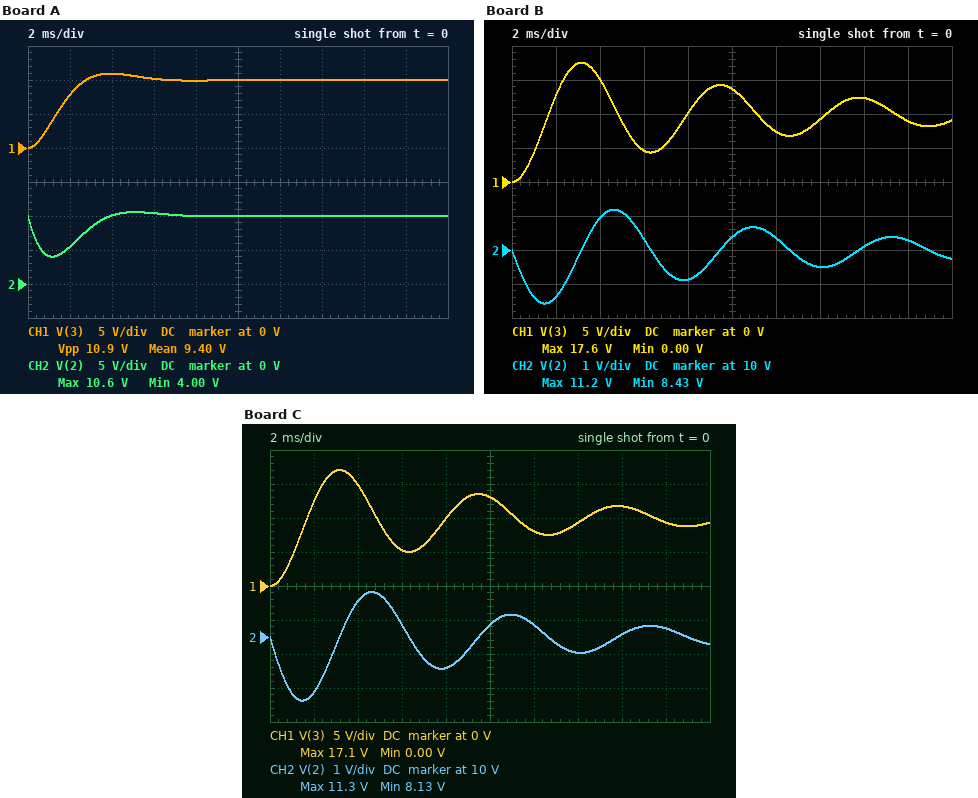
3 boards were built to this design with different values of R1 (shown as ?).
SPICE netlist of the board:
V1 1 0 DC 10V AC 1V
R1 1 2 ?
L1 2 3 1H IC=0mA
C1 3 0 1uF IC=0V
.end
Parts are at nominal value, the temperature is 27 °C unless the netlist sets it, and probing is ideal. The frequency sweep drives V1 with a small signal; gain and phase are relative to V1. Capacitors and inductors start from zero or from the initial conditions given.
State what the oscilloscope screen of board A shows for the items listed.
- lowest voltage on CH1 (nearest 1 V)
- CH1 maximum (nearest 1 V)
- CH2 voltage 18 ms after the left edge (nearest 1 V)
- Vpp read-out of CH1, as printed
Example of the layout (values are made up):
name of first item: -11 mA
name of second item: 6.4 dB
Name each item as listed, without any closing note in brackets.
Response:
lowest voltage on CH1: 0 V
CH1 maximum: 11 V
CH2 voltage 18 ms after the left edge: 10 V
Vpp read-out of CH1, as printed: 10.9 V
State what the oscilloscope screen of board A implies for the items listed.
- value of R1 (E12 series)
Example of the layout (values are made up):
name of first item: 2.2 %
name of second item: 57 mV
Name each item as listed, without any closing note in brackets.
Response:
value of R1: 1.2 kΩ
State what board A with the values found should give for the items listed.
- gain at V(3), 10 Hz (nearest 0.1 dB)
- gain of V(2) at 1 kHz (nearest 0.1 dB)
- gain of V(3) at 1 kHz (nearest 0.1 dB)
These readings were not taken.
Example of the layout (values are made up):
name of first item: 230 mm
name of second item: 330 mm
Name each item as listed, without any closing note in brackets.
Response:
gain at V(3), 10 Hz: 0 dB
gain of V(2) at 1 kHz: -0.2 dB
gain of V(3) at 1 kHz: -31.9 dB
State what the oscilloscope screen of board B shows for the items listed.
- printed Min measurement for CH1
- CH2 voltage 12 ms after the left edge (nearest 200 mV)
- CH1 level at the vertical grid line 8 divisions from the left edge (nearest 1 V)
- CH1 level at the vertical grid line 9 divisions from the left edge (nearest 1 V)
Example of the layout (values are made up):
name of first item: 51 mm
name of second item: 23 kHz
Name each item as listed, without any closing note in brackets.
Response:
printed Min measurement for CH1: 0.00 V
CH2 voltage 12 ms after the left edge: 10.4 V
CH1 level at the vertical grid line 8 divisions from the left edge: 12 V
CH1 level at the vertical grid line 9 divisions from the left edge: 9 V
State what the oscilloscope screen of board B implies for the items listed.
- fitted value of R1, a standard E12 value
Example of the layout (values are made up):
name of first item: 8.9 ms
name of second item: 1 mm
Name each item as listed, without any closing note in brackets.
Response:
fitted value of R1, a standard E12 value: 180 Ω
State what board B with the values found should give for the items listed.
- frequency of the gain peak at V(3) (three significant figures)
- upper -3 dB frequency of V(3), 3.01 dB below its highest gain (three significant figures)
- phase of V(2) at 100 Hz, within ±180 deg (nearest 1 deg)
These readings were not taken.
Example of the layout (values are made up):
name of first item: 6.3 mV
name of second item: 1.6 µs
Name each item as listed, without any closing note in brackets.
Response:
frequency of the gain peak at V(3): 158 Hz
upper -3 dB frequency of V(3), 3.01 dB below its highest gain: 172 Hz
phase of V(2) at 100 Hz, within ±180 deg: -11 deg
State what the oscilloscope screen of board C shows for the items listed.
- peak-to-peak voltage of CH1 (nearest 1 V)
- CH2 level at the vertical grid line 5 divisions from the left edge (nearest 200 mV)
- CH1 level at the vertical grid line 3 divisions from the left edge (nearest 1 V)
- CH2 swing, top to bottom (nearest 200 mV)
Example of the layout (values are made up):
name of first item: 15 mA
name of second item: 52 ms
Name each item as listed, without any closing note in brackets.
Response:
peak-to-peak voltage of CH1: 17 V
CH2 level at the vertical grid line 5 divisions from the left edge: 10.4 V
CH1 level at the vertical grid line 3 divisions from the left edge: 5 V
CH2 swing, top to bottom: 3.2 V
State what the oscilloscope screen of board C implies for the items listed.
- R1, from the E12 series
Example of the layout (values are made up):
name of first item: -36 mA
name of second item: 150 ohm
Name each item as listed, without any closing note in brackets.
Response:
R1, from the E12 series: 220 Ω
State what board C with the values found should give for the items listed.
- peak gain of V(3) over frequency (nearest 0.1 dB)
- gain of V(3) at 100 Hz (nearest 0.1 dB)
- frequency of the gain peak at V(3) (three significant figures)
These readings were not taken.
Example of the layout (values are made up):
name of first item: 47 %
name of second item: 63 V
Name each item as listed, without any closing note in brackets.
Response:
peak gain of V(3) over frequency: 13.2 dB
gain of V(3) at 100 Hz: 4.1 dB
frequency of the gain peak at V(3): 157 Hz
